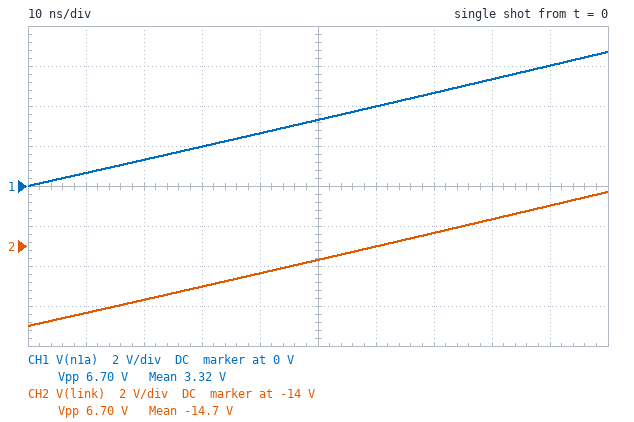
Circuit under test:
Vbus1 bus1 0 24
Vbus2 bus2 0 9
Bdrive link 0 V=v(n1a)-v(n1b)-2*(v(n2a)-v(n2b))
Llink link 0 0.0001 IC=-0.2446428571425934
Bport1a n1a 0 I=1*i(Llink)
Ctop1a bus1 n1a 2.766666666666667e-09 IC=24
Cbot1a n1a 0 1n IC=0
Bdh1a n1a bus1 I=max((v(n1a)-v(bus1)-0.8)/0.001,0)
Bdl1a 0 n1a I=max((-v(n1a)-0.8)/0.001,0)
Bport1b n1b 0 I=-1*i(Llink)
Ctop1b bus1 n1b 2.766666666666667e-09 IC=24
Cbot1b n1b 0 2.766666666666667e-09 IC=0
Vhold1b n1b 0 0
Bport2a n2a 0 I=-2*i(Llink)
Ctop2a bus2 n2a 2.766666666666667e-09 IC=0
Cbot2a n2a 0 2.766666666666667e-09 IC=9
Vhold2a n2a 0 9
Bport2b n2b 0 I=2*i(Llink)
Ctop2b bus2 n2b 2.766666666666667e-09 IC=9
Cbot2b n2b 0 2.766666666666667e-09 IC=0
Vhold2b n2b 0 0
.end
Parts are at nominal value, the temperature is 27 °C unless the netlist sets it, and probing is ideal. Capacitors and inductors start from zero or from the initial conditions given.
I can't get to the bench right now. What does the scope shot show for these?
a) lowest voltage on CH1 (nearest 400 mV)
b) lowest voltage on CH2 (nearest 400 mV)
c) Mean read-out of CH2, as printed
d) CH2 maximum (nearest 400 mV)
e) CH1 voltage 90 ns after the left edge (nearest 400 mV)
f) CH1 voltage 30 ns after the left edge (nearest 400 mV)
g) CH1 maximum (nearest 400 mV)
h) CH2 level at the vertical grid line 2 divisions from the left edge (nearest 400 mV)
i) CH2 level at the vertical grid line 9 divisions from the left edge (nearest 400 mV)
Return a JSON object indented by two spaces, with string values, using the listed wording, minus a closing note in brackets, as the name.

{
  "lowest voltage on CH1": "0 V",
  "lowest voltage on CH2": "-18.0 V",
  "Mean read-out of CH2, as printed": "-14.7 V",
  "CH2 maximum": "-11.2 V",
  "CH1 voltage 90 ns after the left edge": "6.0 V",
  "CH1 voltage 30 ns after the left edge": "2.0 V",
  "CH1 maximum": "6.8 V",
  "CH2 level at the vertical grid line 2 divisions from the left edge": "-16.8 V",
  "CH2 level at the vertical grid line 9 divisions from the left edge": "-12.0 V"
}
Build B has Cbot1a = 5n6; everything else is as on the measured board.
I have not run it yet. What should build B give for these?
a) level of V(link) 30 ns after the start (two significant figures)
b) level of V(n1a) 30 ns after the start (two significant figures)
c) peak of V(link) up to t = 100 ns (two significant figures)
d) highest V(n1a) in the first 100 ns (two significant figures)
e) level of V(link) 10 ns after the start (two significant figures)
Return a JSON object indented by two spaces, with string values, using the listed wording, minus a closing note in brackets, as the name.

{
  "level of V(link) 30 ns after the start": "-17 V",
  "level of V(n1a) 30 ns after the start": "890 mV",
  "peak of V(link) up to t = 100 ns": "-15 V",
  "highest V(n1a) in the first 100 ns": "3.0 V",
  "level of V(link) 10 ns after the start": "-18 V"
}
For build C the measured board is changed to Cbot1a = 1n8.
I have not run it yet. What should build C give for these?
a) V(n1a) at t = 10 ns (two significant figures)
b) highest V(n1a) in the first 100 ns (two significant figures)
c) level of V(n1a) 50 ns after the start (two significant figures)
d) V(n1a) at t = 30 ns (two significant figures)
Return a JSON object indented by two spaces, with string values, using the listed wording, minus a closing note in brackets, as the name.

{
  "V(n1a) at t = 10 ns": "540 mV",
  "highest V(n1a) in the first 100 ns": "5.5 V",
  "level of V(n1a) 50 ns after the start": "2.7 V",
  "V(n1a) at t = 30 ns": "1.6 V"
}
